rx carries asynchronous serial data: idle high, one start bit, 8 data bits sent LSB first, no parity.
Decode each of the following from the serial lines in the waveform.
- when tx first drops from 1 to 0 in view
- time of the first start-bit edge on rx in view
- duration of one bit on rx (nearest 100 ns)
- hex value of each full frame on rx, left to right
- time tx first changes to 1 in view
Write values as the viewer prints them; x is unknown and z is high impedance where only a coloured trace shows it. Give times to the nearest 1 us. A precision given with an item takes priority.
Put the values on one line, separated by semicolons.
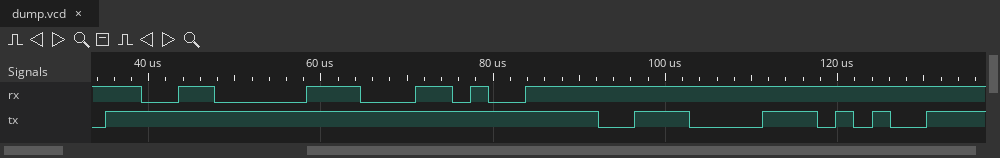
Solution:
92 us; 39 us; 2100 ns; 06, 2C; 35 us
